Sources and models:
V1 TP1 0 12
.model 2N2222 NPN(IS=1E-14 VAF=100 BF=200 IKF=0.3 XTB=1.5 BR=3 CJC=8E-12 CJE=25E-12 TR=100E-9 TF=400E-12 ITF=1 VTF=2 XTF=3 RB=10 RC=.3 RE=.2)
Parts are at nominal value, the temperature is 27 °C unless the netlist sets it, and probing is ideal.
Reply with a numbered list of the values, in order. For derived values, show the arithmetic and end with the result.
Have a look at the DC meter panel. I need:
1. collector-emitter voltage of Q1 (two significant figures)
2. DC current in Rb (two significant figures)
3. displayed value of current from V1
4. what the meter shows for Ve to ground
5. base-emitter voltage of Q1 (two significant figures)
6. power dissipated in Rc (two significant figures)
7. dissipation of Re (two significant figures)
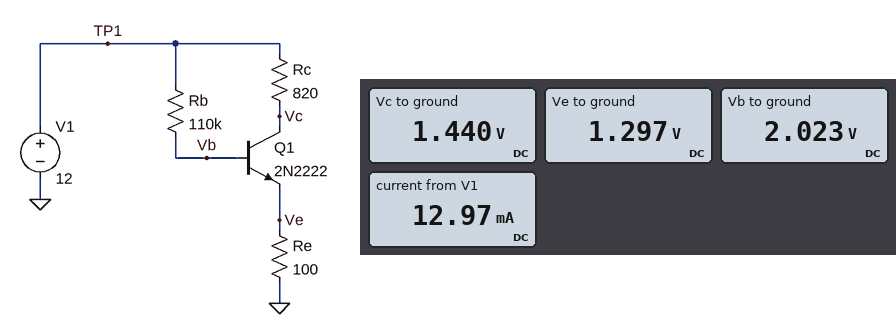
1. 1.44 V - 1.297 V = 140 mV
2. (12 V - 2.023 V) / 110 kΩ = 91 µA
3. 12.97 mA
4. 1.297 V
5. 2.023 V - 1.297 V = 730 mV
6. (12 V - 1.44 V)^2 / 820 Ω = 140 mW
7. (1.297 V)^2 / 100 Ω = 17 mW
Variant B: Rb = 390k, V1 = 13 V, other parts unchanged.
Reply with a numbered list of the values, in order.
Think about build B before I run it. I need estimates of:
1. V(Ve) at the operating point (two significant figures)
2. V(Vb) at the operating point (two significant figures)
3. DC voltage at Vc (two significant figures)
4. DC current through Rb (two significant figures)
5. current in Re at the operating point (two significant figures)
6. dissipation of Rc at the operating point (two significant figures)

1. 630 mV
2. 1.3 V
3. 7.9 V
4. 30 µA
5. 6.3 mA
6. 32 mW
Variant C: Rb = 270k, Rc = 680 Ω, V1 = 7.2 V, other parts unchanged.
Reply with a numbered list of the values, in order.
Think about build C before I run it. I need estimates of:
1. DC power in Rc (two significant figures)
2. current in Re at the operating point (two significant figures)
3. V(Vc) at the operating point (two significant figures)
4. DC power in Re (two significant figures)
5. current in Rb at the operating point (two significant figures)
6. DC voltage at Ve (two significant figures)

1. 14 mW
2. 4.6 mA
3. 4.1 V
4. 2.1 mW
5. 22 µA
6. 460 mV
